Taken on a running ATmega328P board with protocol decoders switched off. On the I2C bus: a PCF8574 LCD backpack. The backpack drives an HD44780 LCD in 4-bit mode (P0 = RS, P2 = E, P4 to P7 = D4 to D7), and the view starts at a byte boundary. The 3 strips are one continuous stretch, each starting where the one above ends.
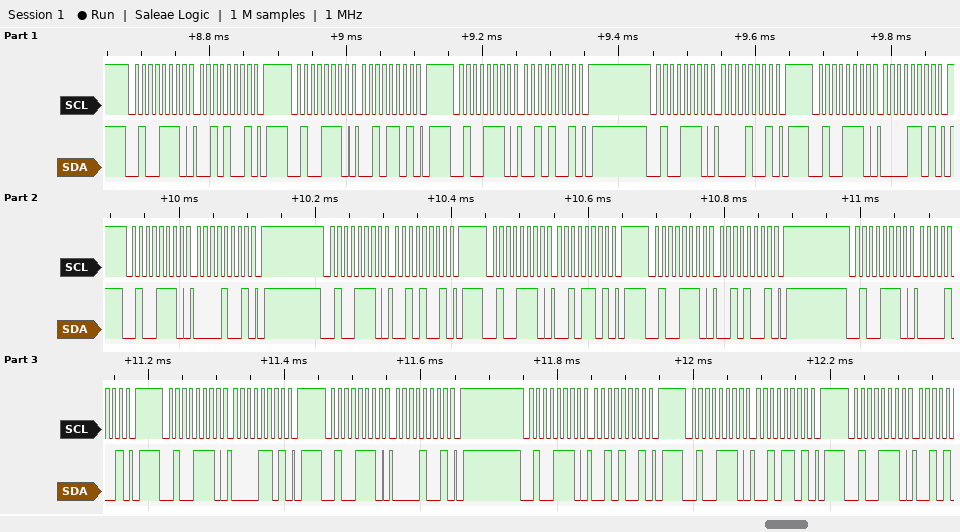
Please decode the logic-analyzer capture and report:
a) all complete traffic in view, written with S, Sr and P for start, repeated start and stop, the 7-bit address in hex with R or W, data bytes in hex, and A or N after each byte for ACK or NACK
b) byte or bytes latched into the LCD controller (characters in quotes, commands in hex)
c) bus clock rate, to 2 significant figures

S 27W A 29 A P S 27W A 2D A P S 27W A 29 A P S 27W A 09 A P S 27W A 0D A P S 27W A 09 A P S 27W A 29 A P S 27W A 2D A P S 27W A 29 A P S 27W A 09 A P S 27W A 0D A P S 27W A 09 A P S 27W A 29 A P S 27W A 2D A P S 27W A
' ' ' '
100 kHz
